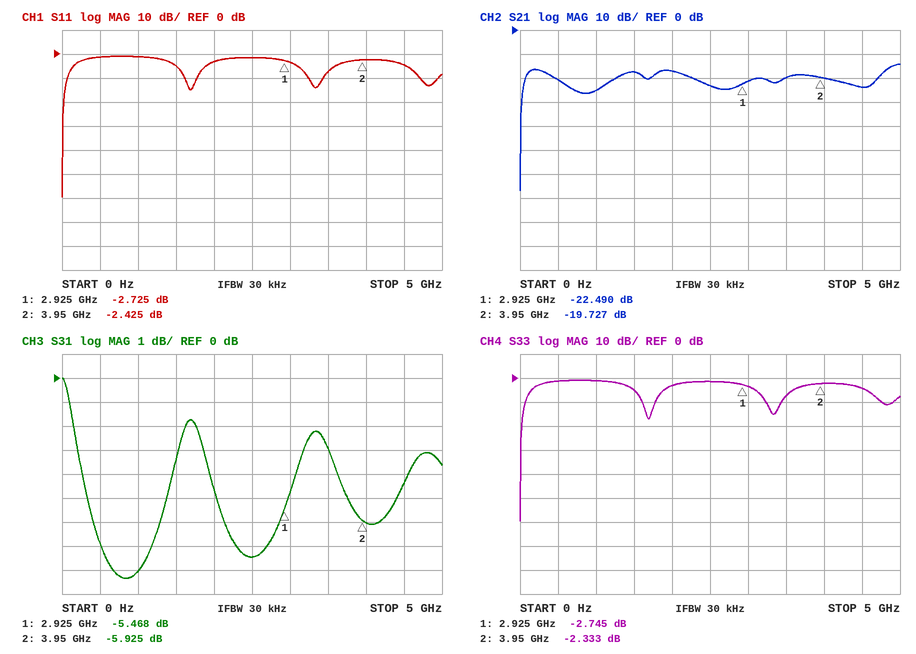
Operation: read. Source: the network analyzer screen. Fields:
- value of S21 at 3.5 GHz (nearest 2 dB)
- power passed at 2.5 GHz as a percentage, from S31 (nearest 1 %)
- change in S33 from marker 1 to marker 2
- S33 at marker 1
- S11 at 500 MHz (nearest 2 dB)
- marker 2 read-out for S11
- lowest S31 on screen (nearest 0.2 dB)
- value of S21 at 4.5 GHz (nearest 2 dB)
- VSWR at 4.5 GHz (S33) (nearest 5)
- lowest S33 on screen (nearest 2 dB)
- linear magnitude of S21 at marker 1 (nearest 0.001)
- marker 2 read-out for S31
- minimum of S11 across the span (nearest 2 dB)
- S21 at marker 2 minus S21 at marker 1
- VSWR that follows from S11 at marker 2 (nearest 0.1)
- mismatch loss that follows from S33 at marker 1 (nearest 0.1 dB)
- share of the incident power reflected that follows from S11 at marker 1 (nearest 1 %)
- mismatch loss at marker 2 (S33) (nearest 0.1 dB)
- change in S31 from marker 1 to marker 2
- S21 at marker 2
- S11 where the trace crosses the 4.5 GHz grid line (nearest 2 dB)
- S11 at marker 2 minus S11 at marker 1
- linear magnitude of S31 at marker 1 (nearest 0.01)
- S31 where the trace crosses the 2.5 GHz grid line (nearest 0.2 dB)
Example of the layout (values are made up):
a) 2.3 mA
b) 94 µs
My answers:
a) -20 dB
b) 18 %
c) 0.412 dB
d) -2.745 dB
e) -2 dB
f) -2.425 dB
g) -8.4 dB
h) -24 dB
i) 5
j) -60 dB
k) 0.075
l) -5.925 dB
m) -60 dB
n) 2.763 dB
o) 7.2
p) 3.3 dB
q) 53 %
r) 3.8 dB
s) -0.457 dB
t) -19.727 dB
u) -4 dB
v) 0.300 dB
w) 0.53
x) -7.4 dB
